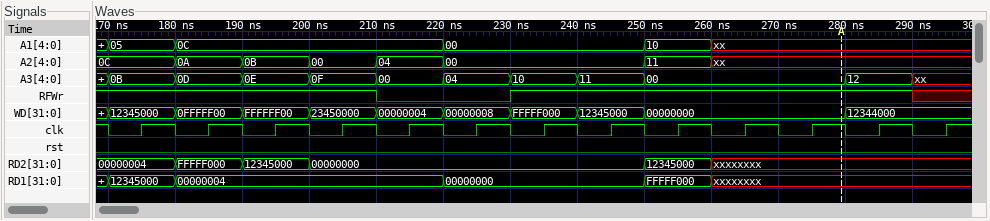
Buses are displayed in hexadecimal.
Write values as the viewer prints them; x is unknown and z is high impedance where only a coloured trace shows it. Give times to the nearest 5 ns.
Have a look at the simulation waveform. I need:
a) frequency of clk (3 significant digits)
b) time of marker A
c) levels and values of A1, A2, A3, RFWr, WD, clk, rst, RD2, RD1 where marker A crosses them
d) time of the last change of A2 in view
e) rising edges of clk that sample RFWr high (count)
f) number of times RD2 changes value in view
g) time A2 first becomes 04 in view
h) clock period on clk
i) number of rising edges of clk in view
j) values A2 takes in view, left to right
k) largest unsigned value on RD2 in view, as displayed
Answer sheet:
100 MHz
280 ns
A1=xx, A2=xx, A3=00, RFWr=1, WD=00000000, clk=1, rst=0, RD2=xxxxxxxx, RD1=xxxxxxxx
260 ns
10
5
210 ns
10 ns
13
0C, 0A, 0B, 00, 04, 00, 11, xx
FFFFF000
